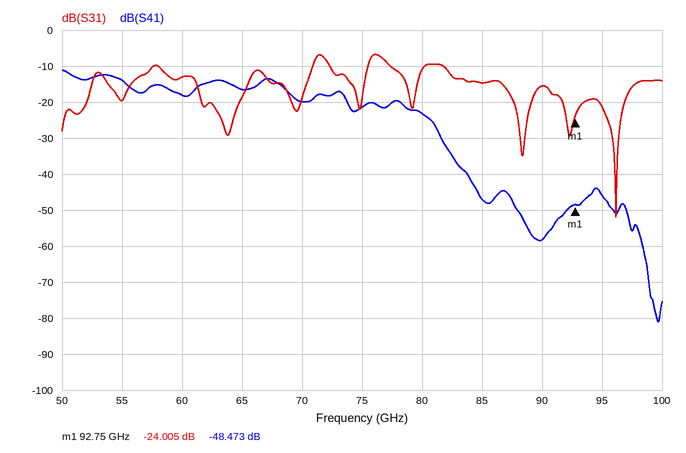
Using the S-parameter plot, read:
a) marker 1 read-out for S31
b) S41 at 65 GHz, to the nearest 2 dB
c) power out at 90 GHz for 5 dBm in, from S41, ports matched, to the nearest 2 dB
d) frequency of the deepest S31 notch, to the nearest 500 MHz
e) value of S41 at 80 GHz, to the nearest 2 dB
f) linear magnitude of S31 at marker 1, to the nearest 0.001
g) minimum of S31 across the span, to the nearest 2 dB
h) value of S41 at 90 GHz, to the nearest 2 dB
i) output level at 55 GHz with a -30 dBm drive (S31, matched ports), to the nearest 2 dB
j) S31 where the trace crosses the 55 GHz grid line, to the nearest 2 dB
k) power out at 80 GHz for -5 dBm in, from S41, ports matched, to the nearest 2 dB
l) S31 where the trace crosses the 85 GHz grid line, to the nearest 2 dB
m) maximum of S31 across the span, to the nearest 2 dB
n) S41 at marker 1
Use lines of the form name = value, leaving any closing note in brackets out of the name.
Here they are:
marker 1 read-out for S31 = -24.005 dB
S41 at 65 GHz, to the nearest 2 dB = -16 dB
power out at 90 GHz for 5 dBm in, from S41, ports matched, to the nearest 2 dB = -54 dBm
frequency of the deepest S31 notch, to the nearest 500 MHz = 96.0 GHz
value of S41 at 80 GHz, to the nearest 2 dB = -24 dB
linear magnitude of S31 at marker 1, to the nearest 0.001 = 0.063
minimum of S31 across the span, to the nearest 2 dB = -52 dB
value of S41 at 90 GHz, to the nearest 2 dB = -58 dB
output level at 55 GHz with a -30 dBm drive (S31, matched ports), to the nearest 2 dB = -50 dBm
S31 where the trace crosses the 55 GHz grid line, to the nearest 2 dB = -20 dB
power out at 80 GHz for -5 dBm in, from S41, ports matched, to the nearest 2 dB = -28 dBm
S31 where the trace crosses the 85 GHz grid line, to the nearest 2 dB = -14 dB
maximum of S31 across the span, to the nearest 2 dB = -6 dB
S41 at marker 1 = -48.473 dB
